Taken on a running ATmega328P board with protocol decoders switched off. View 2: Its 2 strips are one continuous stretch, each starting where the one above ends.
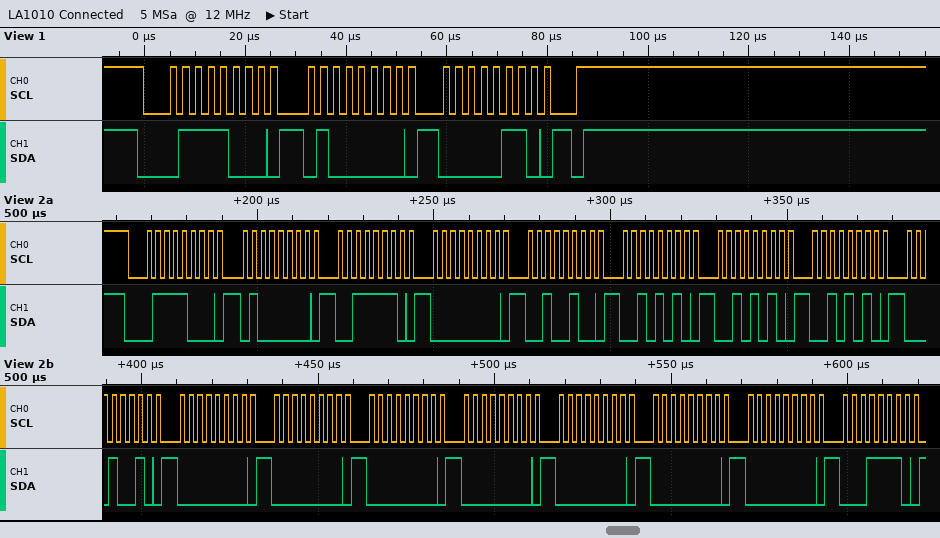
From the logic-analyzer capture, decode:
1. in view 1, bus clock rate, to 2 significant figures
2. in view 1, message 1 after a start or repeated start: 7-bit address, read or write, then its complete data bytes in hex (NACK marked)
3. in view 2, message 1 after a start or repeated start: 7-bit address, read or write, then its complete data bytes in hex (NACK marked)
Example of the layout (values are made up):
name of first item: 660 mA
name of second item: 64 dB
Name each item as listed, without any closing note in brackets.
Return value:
in view 1, bus clock rate, to 2 significant figures: 400 kHz
in view 1, message 1 after a start or repeated start: 7-bit address, read or write, then its complete data bytes in hex: 0x3C write: 40 06
in view 2, message 1 after a start or repeated start: 7-bit address, read or write, then its complete data bytes in hex: 0x3C write: 40 3E 00 24 2A 2A 2A 12 00 00 00 00 00 00 00 1E
